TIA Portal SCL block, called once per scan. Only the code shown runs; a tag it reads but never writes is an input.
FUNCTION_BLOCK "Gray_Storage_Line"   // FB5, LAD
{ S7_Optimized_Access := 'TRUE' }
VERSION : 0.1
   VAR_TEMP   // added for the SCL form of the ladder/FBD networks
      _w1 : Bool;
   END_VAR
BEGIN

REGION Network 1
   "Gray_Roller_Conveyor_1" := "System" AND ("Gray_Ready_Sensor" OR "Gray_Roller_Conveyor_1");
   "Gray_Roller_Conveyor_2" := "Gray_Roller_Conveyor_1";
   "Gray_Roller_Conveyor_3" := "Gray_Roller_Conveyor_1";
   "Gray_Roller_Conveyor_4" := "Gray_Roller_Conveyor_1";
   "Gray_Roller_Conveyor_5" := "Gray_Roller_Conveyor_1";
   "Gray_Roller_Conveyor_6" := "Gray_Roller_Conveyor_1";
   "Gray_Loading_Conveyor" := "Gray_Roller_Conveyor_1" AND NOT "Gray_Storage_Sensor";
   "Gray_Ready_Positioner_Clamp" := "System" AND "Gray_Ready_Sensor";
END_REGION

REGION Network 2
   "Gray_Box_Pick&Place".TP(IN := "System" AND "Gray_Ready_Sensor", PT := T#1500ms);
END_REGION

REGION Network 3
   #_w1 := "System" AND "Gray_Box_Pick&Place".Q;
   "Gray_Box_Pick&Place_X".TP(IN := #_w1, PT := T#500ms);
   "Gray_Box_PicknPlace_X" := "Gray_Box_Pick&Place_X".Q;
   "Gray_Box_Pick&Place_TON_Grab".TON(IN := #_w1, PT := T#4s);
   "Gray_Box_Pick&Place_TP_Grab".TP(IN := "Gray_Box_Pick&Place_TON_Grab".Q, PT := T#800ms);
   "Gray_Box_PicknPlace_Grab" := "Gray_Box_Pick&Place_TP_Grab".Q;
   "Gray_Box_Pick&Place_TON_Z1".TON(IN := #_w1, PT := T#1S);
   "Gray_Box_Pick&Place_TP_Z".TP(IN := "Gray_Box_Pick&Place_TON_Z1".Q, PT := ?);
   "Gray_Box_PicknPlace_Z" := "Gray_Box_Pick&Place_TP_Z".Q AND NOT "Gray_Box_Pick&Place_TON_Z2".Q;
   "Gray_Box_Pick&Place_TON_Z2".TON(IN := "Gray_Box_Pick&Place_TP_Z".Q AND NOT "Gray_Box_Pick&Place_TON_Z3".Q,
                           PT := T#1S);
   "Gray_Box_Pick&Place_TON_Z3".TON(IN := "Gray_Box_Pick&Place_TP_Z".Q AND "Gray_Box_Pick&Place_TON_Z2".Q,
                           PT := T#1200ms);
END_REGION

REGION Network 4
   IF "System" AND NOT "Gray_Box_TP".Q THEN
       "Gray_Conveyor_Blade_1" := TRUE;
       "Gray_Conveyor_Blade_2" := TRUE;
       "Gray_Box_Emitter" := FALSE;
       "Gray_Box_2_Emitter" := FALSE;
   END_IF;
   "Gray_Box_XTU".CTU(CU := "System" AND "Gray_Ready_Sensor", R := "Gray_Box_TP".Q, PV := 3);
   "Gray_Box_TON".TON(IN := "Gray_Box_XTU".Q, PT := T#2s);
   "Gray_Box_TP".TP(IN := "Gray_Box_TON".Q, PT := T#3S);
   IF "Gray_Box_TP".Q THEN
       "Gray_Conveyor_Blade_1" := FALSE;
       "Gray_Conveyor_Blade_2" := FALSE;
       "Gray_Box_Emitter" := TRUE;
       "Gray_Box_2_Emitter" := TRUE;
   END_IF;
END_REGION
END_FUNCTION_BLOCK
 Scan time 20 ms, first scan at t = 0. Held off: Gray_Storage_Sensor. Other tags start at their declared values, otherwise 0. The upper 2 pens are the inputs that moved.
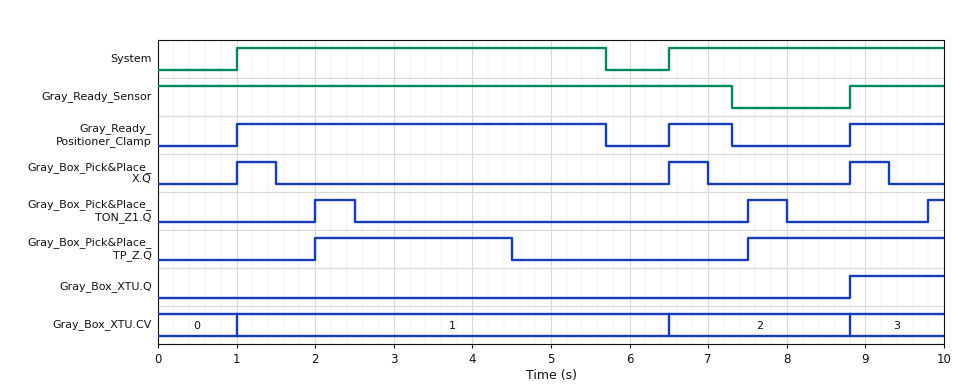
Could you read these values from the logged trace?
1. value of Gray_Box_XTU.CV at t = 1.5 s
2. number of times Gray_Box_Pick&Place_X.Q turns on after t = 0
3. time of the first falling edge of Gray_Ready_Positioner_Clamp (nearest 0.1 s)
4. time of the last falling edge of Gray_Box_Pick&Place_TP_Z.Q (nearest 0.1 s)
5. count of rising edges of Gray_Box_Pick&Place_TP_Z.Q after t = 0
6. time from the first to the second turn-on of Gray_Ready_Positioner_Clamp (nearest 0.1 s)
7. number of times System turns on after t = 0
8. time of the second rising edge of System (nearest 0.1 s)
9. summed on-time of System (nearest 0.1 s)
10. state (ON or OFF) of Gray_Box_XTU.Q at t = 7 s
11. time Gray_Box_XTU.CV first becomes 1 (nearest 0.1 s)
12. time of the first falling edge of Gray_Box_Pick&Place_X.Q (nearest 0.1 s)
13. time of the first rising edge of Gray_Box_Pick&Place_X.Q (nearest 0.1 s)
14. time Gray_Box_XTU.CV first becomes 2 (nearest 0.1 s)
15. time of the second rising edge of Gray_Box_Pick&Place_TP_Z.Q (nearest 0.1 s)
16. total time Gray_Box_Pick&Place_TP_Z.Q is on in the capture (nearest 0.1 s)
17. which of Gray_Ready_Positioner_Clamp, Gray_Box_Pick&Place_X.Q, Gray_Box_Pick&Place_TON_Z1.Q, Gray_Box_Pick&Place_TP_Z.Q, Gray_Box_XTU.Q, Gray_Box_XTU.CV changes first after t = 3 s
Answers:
1
3
5.7 s
4.5 s
2
5.5 s
2
6.5 s
8.2 s
OFF
1.0 s
1.5 s
1.0 s
6.5 s
7.5 s
5.0 s
Gray_Box_Pick&Place_TP_Z.Q
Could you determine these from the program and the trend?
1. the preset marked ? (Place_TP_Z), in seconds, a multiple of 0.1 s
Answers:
2.5 s
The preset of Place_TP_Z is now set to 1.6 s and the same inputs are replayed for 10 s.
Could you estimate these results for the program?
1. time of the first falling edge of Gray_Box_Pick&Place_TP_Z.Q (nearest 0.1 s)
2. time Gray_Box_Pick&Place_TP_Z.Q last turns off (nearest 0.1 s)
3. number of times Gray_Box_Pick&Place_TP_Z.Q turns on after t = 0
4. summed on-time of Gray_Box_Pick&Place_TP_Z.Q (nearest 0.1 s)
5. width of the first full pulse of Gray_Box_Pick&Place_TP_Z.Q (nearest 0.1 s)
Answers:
3.6 s
9.1 s
3
3.4 s
1.6 s
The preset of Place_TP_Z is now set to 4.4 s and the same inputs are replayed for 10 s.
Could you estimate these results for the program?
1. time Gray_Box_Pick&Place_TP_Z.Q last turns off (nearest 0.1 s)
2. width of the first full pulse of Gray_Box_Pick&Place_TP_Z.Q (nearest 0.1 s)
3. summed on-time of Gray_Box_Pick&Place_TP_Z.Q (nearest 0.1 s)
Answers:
6.4 s
4.4 s
6.9 s
